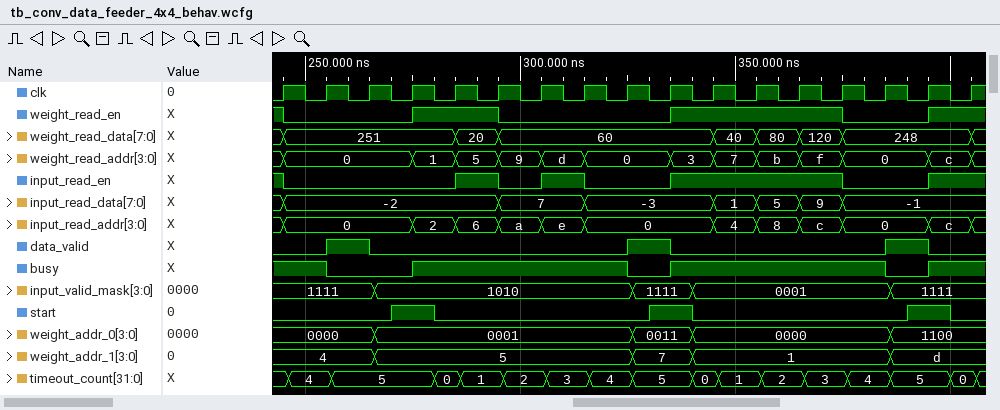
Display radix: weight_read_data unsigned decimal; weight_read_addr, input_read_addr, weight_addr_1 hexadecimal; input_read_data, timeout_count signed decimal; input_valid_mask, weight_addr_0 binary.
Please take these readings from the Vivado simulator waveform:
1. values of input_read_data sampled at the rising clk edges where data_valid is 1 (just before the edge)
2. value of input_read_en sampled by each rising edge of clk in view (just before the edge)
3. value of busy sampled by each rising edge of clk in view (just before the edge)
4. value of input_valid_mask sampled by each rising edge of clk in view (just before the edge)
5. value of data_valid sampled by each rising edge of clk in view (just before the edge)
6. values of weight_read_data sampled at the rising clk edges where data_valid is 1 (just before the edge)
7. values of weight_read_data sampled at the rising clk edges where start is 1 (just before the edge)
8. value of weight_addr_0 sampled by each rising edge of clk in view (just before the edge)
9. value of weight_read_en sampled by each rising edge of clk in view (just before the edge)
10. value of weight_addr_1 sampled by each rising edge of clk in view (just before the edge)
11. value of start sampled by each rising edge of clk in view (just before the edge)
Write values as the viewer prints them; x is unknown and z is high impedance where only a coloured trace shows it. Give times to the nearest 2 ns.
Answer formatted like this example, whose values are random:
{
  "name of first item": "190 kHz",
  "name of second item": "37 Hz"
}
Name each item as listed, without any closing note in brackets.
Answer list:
{
  "values of input_read_data sampled at the rising clk edges where data_valid is 1": "-2, -3, -1",
  "value of input_read_en sampled by each rising edge of clk in view": "1 0 0 0 0 1 0 1 0 0 1 1 1 1 0 0 1",
  "value of busy sampled by each rising edge of clk in view": "1 1 0 0 1 1 1 1 1 0 1 1 1 1 1 0 1",
  "value of input_valid_mask sampled by each rising edge of clk in view": "1111, 1111, 1111, 1010, 1010, 1010, 1010, 1010, 1010, 1111, 0001, 0001, 0001, 0001, 0001, 1111, 1111",
  "value of data_valid sampled by each rising edge of clk in view": "0 0 1 0 0 0 0 0 0 1 0 0 0 0 0 1 0",
  "values of weight_read_data sampled at the rising clk edges where data_valid is 1": "251, 60, 248",
  "values of weight_read_data sampled at the rising clk edges where start is 1": "251, 60, 248",
  "value of weight_addr_0 sampled by each rising edge of clk in view": "0000, 0000, 0000, 0001, 0001, 0001, 0001, 0001, 0001, 0011, 0000, 0000, 0000, 0000, 0000, 1100, 1100",
  "value of weight_read_en sampled by each rising edge of clk in view": "1 0 0 0 1 1 0 0 0 0 1 1 1 1 0 0 1",
  "value of weight_addr_1 sampled by each rising edge of clk in view": "4, 4, 4, 5, 5, 5, 5, 5, 5, 7, 1, 1, 1, 1, 1, d, d",
  "value of start sampled by each rising edge of clk in view": "0 0 0 1 0 0 0 0 0 1 0 0 0 0 0 1 0"
}
